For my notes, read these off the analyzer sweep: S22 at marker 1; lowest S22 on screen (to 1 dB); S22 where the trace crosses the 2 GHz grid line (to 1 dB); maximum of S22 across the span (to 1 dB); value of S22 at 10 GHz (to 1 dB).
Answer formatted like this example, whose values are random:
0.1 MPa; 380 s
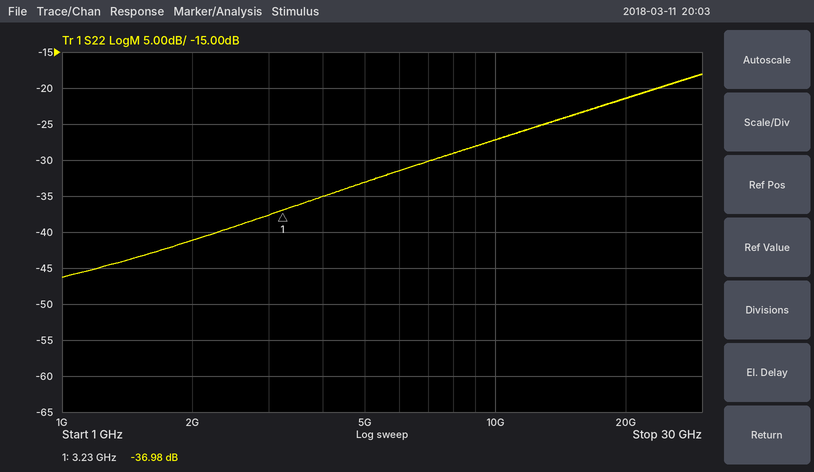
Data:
-36.98 dB; -46 dB; -41 dB; -18 dB; -27 dB
